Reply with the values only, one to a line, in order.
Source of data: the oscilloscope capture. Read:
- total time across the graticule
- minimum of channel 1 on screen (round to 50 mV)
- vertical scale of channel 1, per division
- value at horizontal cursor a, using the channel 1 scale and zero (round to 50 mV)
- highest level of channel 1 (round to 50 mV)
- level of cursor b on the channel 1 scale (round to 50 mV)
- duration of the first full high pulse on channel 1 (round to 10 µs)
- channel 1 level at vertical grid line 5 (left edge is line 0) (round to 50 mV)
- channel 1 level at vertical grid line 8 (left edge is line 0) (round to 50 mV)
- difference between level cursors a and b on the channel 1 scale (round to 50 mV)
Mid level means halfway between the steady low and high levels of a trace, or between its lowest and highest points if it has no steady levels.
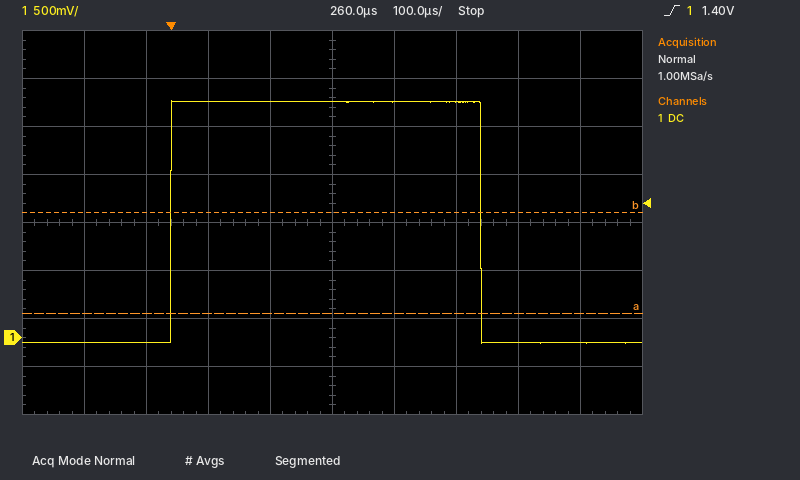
1 ms
-50 mV
500 mV
250 mV
2.45 V
1.30 V
500 µs
2.45 V
-50 mV
1.05 V
